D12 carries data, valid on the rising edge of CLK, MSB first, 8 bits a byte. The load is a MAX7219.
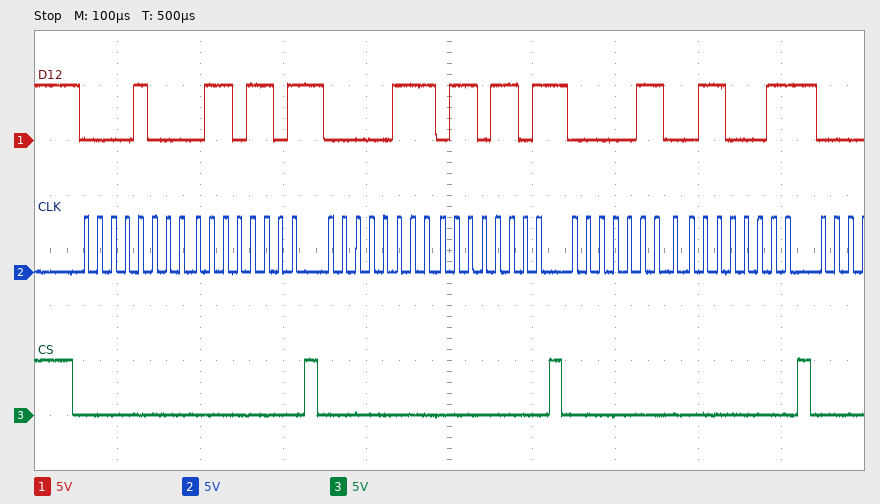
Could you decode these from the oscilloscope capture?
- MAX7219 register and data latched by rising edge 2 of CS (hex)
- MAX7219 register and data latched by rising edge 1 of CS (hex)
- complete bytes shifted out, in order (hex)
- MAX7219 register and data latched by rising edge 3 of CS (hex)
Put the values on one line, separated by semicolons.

register 0x7, data 0x6D; register 0x8, data 0x6D; 08 6D 07 6D 06 63; register 0x6, data 0x63
